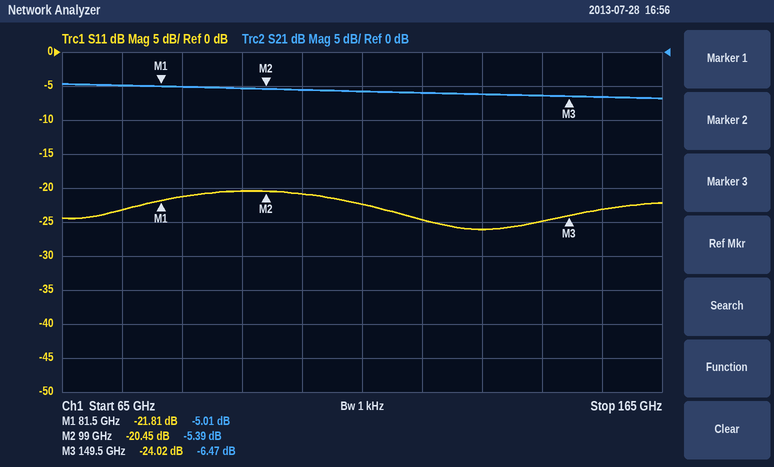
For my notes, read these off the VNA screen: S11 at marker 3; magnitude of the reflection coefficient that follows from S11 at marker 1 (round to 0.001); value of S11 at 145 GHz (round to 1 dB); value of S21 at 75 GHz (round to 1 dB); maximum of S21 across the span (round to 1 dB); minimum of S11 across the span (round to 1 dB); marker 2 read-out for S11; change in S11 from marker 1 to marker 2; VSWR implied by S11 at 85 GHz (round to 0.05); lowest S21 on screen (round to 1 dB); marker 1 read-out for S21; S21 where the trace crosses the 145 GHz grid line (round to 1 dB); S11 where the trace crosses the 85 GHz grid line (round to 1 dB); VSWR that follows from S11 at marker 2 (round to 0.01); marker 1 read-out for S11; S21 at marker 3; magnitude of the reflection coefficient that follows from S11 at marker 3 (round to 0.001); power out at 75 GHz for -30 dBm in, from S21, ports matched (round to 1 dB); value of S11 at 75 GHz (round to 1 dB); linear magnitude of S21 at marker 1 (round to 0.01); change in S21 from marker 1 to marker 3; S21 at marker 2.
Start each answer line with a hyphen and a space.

- -24.02 dB
- 0.081
- -25 dB
- -5 dB
- -5 dB
- -26 dB
- -20.45 dB
- 1.36 dB
- 1.20
- -7 dB
- -5.01 dB
- -6 dB
- -21 dB
- 1.21
- -21.81 dB
- -6.47 dB
- 0.063
- -35 dBm
- -23 dB
- 0.56
- -1.46 dB
- -5.39 dB
